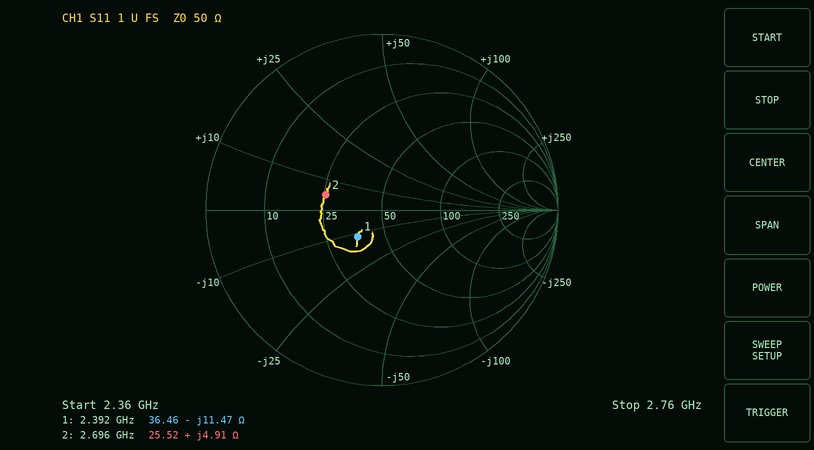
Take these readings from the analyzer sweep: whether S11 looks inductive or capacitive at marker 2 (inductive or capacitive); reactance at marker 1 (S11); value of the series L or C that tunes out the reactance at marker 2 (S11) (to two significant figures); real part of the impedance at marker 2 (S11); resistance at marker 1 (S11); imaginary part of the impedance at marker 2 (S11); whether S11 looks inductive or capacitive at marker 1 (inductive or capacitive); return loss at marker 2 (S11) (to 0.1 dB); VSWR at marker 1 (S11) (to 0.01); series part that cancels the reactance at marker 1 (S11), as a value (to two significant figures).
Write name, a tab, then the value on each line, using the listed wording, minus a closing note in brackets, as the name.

whether S11 looks inductive or capacitive at marker 2	inductive
reactance at marker 1	-11.47 Ω
value of the series L or C that tunes out the reactance at marker 2 (S11)	12 pF
real part of the impedance at marker 2	25.52 Ω
resistance at marker 1	36.46 Ω
imaginary part of the impedance at marker 2	+4.91 Ω
whether S11 looks inductive or capacitive at marker 1	capacitive
return loss at marker 2 (S11)	9.6 dB
VSWR at marker 1 (S11)	1.51
series part that cancels the reactance at marker 1 (S11), as a value	760 pH
